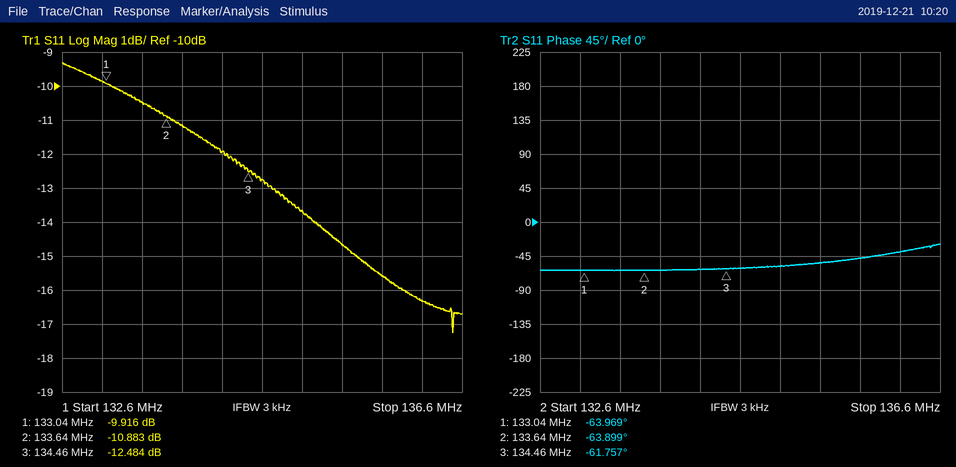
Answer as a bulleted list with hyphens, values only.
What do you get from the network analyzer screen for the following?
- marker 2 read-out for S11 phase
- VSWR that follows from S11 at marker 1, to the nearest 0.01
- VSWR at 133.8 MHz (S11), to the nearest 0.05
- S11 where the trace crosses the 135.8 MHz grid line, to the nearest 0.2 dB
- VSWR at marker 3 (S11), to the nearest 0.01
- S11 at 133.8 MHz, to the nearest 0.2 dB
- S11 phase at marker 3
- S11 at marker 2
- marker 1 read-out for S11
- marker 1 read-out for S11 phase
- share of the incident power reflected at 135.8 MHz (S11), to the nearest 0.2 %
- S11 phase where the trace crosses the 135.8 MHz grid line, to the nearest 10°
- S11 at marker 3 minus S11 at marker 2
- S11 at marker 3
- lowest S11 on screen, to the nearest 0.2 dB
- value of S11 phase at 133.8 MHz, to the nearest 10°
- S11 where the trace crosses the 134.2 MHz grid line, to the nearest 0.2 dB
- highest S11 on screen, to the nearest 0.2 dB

- -63.899°
- 1.94
- 1.75
- -15.6 dB
- 1.62
- -11.2 dB
- -61.757°
- -10.883 dB
- -9.916 dB
- -63.969°
- 2.8 %
- -50°
- -1.601 dB
- -12.484 dB
- -17.2 dB
- -60°
- -12.0 dB
- -9.4 dB
